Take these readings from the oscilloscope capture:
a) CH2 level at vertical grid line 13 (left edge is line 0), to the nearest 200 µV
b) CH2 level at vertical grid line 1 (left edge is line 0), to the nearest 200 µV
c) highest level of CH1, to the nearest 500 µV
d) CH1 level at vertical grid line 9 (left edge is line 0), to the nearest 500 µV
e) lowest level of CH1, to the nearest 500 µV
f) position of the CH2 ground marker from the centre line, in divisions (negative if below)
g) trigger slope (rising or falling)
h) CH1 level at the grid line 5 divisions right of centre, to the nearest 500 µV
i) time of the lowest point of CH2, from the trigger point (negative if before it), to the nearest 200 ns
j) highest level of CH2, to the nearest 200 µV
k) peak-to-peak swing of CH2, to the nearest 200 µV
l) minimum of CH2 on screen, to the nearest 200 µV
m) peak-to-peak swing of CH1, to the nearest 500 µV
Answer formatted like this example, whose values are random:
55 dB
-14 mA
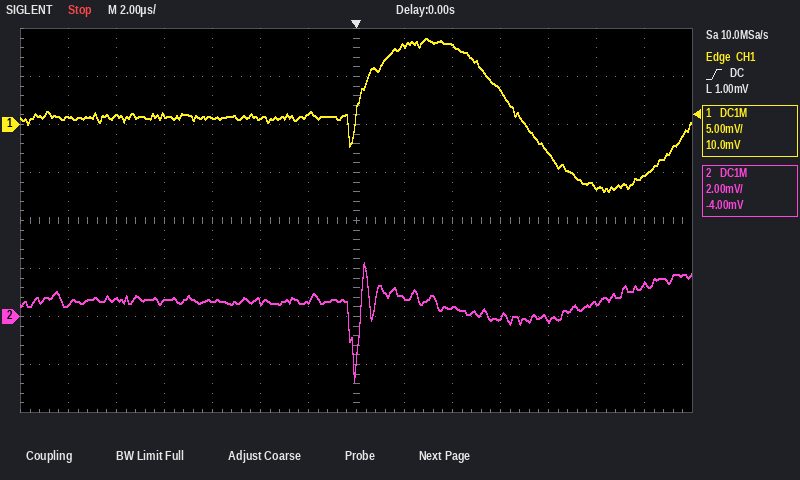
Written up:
1.4 mV
400 µV
9.0 mV
8.5 mV
-7.0 mV
-2.0 div
rising
-6.5 mV
0.0 µs
2.2 mV
5.0 mV
-2.8 mV
16.0 mV
